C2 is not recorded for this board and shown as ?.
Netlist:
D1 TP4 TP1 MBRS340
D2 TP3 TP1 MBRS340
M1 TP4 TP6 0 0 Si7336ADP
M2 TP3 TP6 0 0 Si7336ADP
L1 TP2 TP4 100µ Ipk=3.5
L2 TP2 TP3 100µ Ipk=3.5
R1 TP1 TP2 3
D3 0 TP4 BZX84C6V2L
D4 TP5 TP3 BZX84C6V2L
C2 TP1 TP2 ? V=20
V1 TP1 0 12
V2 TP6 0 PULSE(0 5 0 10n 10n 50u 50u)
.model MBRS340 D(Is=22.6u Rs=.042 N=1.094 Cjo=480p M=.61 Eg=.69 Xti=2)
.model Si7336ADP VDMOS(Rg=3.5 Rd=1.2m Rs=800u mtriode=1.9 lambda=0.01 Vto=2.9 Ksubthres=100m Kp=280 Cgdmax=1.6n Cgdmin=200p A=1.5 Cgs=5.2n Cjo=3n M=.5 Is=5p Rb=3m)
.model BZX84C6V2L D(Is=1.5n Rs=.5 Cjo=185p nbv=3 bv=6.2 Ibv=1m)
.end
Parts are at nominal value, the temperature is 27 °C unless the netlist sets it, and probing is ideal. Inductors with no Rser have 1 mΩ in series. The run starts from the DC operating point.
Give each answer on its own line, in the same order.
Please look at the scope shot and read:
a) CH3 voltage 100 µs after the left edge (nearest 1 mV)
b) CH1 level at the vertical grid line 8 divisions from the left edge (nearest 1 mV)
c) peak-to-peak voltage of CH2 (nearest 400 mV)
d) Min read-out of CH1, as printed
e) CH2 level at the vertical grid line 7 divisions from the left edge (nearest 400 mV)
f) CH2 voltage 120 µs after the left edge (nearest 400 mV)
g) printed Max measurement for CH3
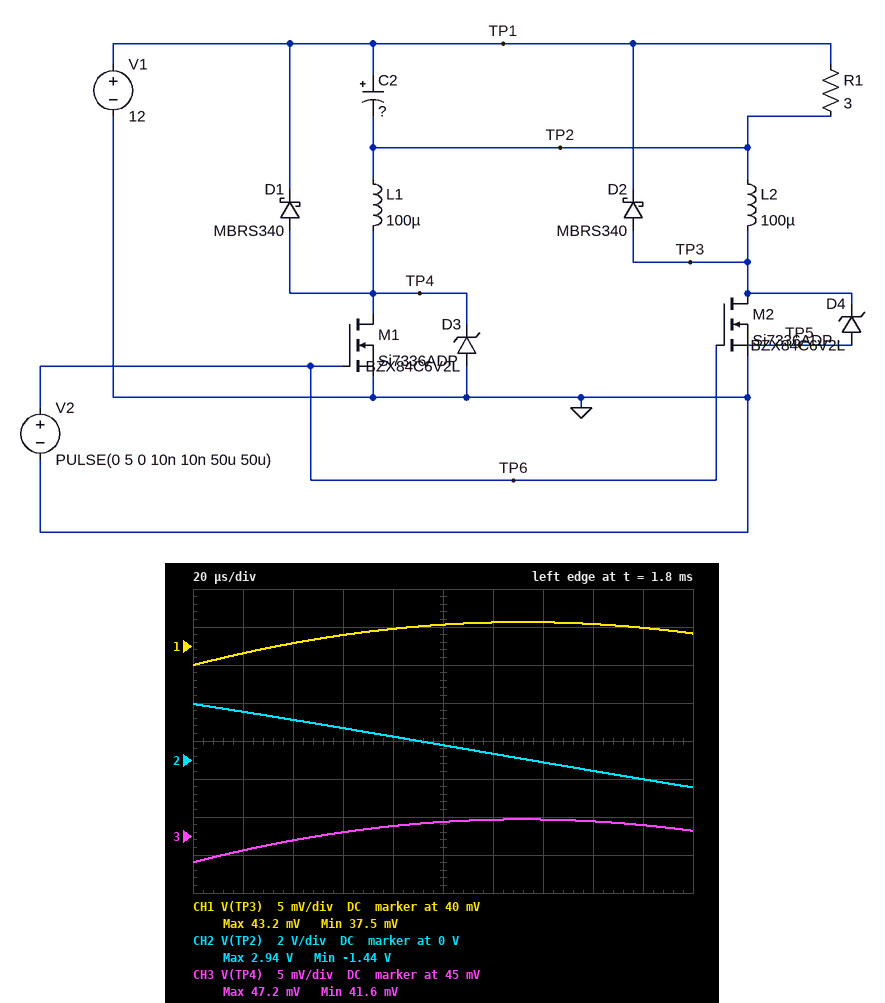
47 mV
43 mV
4.4 V
37.5 mV
0 V
400 mV
47.2 mV
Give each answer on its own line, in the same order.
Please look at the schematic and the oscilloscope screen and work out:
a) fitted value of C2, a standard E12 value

1.2 mF
